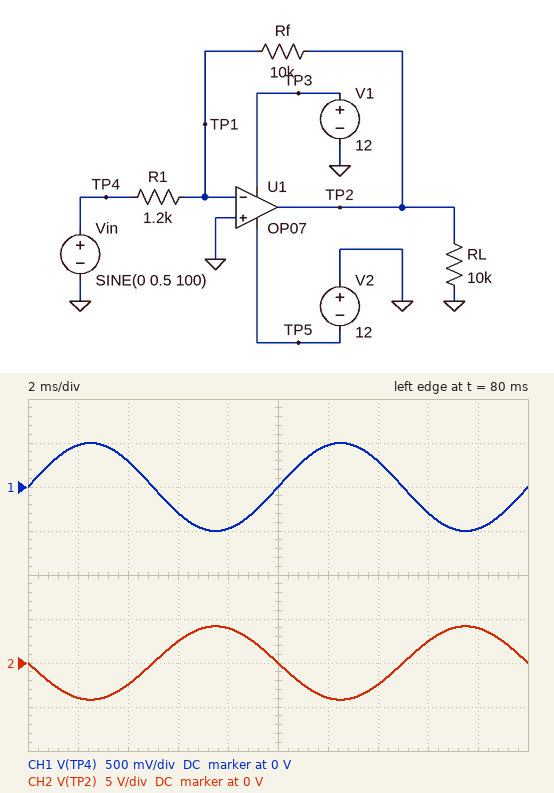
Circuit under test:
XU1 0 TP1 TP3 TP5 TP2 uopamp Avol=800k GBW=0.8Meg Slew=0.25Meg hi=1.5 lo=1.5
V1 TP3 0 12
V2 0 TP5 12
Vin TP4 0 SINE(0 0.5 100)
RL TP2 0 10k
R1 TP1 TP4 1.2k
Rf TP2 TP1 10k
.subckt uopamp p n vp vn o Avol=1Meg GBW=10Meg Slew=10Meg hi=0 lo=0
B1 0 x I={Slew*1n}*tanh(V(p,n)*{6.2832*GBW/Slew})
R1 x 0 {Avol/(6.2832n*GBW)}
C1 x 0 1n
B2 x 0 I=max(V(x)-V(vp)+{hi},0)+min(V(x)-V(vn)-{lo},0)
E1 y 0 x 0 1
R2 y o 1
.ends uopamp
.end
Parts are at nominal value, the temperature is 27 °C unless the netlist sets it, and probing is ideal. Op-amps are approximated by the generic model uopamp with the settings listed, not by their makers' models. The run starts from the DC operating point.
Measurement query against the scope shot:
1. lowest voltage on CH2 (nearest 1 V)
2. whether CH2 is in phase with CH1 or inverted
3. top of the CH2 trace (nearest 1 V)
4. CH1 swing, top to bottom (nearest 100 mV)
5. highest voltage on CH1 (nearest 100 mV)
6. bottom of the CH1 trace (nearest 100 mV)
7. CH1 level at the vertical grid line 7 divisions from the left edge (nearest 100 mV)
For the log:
-4 V
inverted
4 V
1.0 V
500 mV
-500 mV
300 mV
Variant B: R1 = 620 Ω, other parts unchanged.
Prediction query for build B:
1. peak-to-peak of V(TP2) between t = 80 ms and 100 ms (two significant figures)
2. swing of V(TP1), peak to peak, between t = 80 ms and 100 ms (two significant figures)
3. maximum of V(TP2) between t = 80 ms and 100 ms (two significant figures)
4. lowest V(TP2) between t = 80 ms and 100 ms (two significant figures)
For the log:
16 V
2.0 mV
8.1 V
-8.1 V
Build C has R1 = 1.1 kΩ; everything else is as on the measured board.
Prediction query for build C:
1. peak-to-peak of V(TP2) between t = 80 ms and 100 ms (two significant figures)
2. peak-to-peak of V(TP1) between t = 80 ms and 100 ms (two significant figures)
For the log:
9.1 V
1.1 mV
